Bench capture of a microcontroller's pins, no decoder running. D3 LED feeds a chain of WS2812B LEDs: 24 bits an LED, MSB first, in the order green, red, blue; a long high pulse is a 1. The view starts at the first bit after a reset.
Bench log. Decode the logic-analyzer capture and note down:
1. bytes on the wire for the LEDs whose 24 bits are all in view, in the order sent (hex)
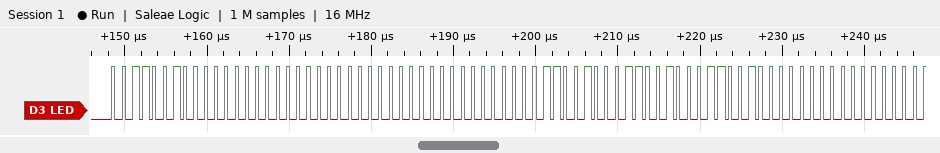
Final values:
32 00 00 00 00 32 32 32 00
